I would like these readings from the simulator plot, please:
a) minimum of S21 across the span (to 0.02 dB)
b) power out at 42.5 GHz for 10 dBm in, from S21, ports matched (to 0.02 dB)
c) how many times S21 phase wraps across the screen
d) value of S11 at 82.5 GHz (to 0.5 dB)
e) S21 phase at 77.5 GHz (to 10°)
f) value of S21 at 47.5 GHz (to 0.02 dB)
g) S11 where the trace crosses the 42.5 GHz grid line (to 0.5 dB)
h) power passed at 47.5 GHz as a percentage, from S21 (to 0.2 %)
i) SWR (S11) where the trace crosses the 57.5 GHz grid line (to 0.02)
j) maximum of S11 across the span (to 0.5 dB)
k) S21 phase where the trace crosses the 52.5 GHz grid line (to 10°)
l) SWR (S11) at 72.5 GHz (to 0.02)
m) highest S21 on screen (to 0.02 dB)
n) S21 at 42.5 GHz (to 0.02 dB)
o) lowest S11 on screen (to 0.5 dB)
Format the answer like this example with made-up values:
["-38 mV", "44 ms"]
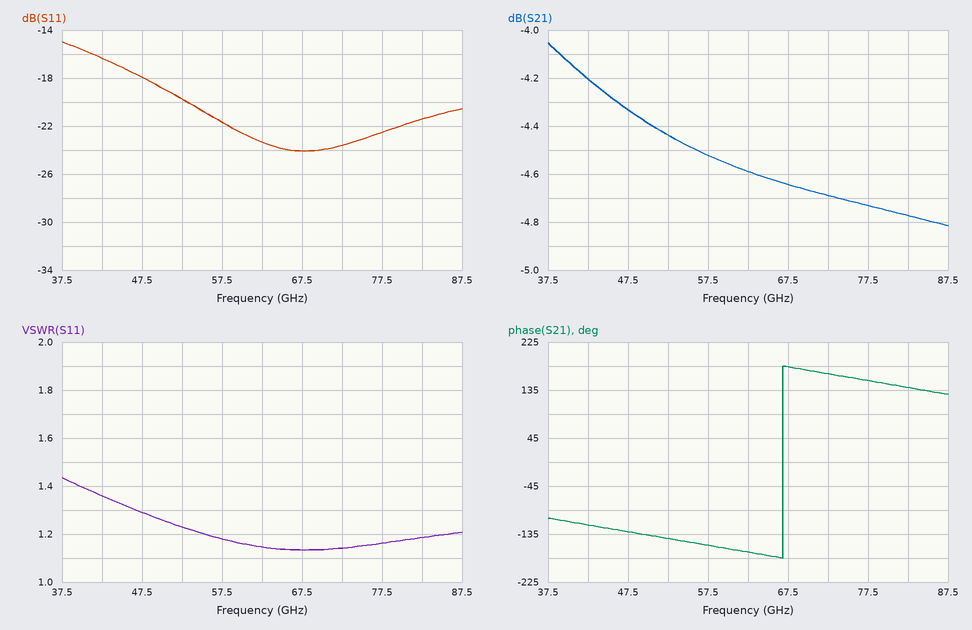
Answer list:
["-4.82 dB", "5.80 dBm", "1", "-21.5 dB", "150°", "-4.34 dB", "-16.5 dB", "36.8 %", "1.18", "-15.0 dB", "-140°", "1.14", "-4.06 dB", "-4.20 dB", "-24.0 dB"]
